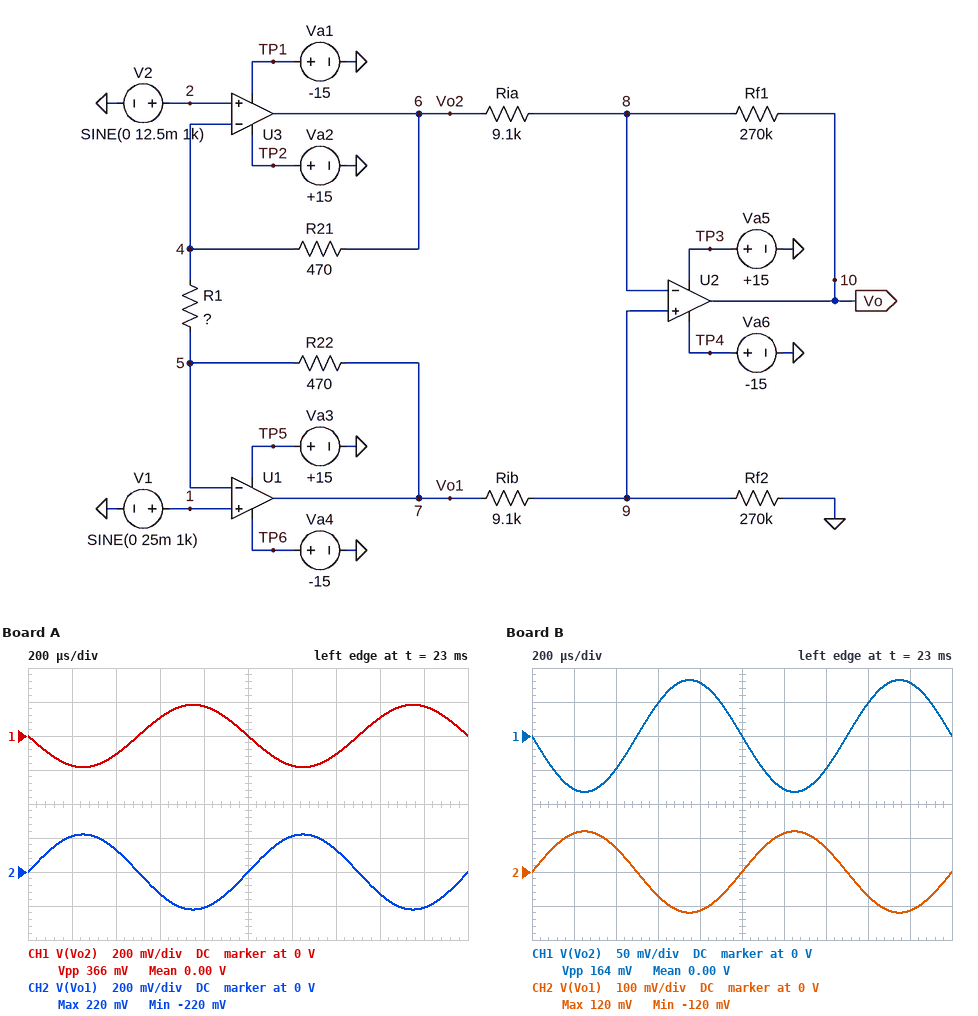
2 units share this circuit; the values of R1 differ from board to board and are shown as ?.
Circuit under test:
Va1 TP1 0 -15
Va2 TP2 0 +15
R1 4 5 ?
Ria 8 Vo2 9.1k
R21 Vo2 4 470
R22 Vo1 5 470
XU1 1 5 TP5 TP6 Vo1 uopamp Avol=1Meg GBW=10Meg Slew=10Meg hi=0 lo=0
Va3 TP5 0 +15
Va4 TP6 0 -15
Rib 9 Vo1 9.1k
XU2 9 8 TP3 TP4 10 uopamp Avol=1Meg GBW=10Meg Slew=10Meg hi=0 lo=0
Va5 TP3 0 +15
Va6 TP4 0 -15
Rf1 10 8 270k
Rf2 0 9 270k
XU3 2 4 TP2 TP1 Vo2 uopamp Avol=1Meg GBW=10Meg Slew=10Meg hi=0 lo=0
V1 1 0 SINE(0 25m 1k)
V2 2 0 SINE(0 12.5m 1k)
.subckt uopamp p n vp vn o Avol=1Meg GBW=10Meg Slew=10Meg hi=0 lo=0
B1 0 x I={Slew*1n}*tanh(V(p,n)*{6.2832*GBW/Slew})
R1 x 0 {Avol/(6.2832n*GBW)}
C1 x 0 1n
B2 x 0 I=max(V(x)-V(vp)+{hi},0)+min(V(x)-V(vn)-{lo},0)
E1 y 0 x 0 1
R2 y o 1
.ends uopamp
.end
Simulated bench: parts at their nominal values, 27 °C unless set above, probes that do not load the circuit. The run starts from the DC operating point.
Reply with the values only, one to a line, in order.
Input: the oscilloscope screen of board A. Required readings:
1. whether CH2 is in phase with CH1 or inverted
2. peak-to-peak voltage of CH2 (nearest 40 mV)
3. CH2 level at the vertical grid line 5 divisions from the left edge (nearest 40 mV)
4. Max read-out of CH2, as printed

inverted
440 mV
0 V
220 mV
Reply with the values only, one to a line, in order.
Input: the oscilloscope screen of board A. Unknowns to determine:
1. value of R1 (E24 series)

30 Ω
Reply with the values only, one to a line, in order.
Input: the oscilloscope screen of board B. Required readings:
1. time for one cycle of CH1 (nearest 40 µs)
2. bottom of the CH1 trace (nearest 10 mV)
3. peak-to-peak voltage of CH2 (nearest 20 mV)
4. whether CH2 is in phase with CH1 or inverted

1.00 ms
-80 mV
240 mV
inverted
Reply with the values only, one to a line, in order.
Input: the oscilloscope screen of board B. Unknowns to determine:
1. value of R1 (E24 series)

62 Ω
